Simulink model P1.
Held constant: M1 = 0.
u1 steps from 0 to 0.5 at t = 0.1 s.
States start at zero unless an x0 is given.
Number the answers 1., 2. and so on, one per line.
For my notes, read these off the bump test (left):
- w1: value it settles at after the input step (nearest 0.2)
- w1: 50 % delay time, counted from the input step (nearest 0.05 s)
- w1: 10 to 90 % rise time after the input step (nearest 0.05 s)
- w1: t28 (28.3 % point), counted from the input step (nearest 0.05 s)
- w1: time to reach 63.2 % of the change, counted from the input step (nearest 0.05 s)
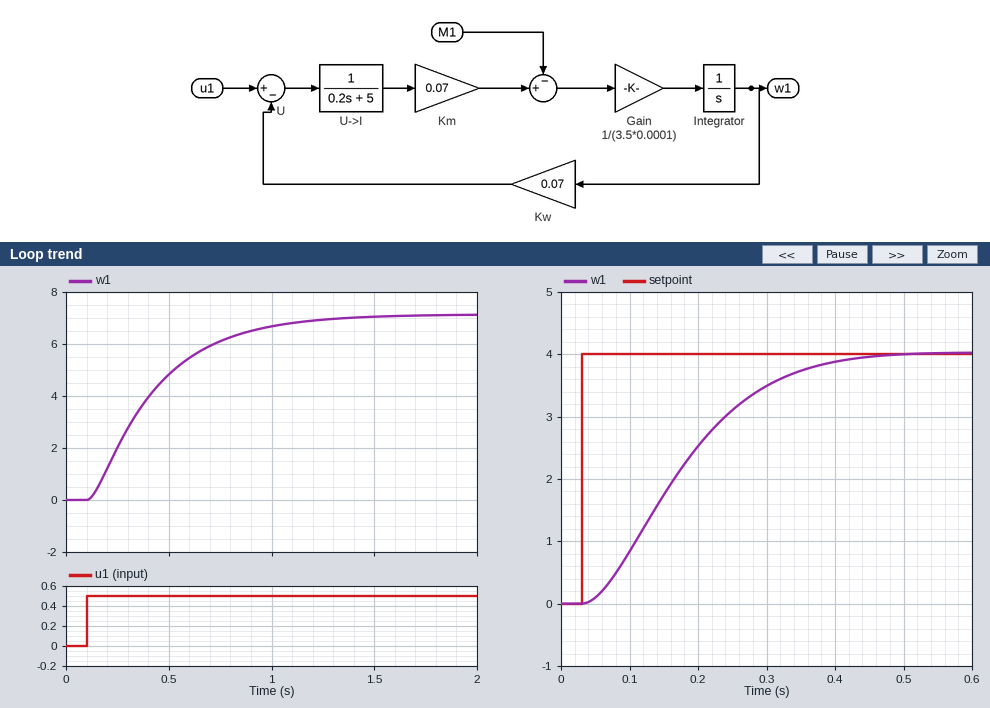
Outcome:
1. 7.2
2. 0.25 s
3. 0.70 s
4. 0.15 s
5. 0.35 s
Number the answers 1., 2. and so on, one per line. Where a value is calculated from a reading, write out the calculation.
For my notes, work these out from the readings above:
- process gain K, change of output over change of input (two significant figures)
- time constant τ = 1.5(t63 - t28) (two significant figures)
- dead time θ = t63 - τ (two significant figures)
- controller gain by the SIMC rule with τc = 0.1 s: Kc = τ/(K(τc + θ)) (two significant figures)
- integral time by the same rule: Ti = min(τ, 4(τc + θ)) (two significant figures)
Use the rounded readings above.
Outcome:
1. (7.2 - 0) / 0.5 = 14
2. 1.5 × (0.35 - 0.15) = 0.30 s
3. 0.35 - 0.3 = 0.050 s
4. 0.3 / (14 × (0.1 + 0.05)) = 0.14
5. min(0.3, 4 × (0.1 + 0.05)) = 0.30 s
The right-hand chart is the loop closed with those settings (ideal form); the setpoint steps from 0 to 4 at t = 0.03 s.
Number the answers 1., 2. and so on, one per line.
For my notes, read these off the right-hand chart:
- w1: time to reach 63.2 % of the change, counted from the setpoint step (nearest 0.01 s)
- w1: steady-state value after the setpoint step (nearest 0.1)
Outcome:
1. 0.17 s
2. 4.0
